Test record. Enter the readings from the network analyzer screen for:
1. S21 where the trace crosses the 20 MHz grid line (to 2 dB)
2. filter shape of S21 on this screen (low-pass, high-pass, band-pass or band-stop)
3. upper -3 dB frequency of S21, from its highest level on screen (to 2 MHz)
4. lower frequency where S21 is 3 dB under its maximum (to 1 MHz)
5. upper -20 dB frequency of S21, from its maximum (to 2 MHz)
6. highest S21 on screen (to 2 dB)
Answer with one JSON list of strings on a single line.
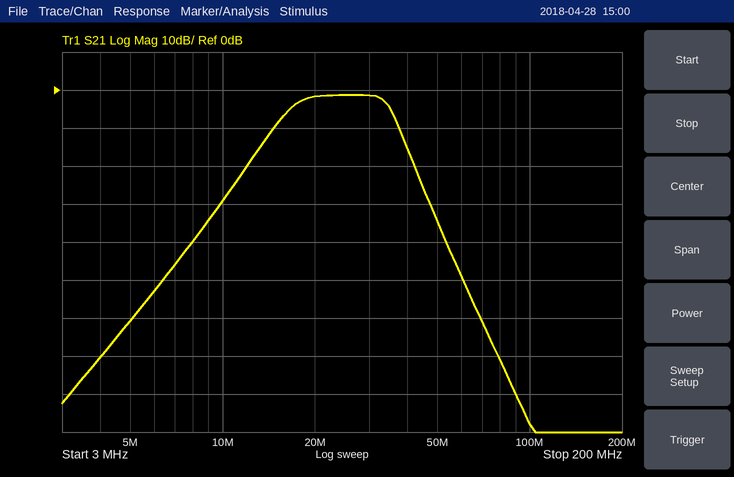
["-2 dB", "band-pass", "34 MHz", "17 MHz", "42 MHz", "-2 dB"]
